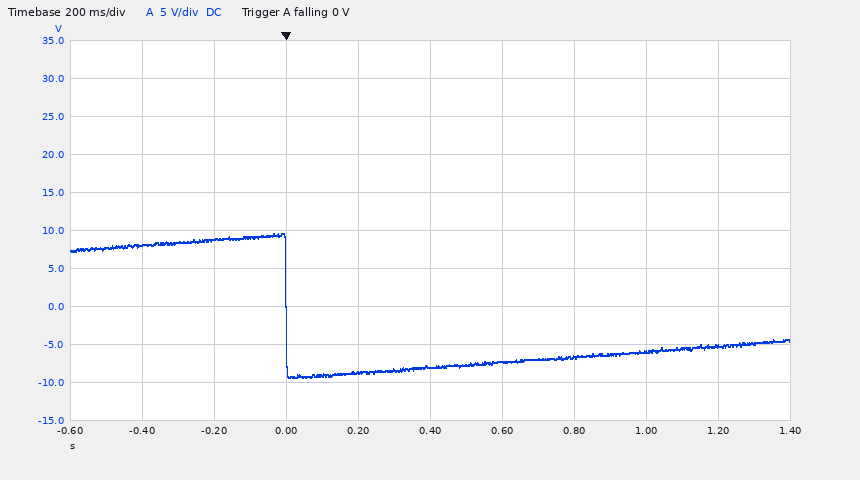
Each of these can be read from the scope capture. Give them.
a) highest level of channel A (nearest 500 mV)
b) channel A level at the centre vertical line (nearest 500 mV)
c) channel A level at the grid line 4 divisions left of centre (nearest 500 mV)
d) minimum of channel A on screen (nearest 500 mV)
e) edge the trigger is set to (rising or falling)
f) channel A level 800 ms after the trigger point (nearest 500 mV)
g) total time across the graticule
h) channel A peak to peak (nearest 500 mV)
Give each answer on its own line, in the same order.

9.5 V
-8.0 V
8.0 V
-9.5 V
falling
-6.5 V
2 s
19.0 V
